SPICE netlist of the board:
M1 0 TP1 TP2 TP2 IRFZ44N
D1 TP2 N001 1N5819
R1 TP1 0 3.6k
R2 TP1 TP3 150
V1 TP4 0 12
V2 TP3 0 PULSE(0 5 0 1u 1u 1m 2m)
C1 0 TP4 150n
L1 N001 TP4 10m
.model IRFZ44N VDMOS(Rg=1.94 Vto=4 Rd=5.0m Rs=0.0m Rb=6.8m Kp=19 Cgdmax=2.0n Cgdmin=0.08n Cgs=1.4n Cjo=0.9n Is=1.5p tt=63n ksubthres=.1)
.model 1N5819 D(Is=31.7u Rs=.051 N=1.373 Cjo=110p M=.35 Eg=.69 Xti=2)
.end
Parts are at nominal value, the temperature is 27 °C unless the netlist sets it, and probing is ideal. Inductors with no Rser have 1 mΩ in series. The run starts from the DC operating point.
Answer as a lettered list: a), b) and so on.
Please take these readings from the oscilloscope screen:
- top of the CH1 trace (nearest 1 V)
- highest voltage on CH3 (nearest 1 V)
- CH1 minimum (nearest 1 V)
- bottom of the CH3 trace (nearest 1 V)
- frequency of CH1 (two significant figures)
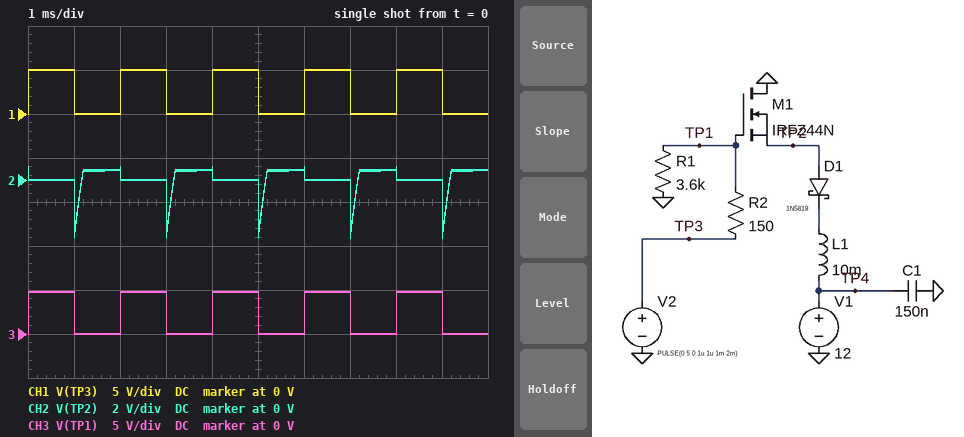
a) 5 V
b) 5 V
c) 0 V
d) 0 V
e) 500 Hz
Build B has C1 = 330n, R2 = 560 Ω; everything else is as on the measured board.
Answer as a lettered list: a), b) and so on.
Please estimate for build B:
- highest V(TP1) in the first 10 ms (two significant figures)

a) 4.3 V
